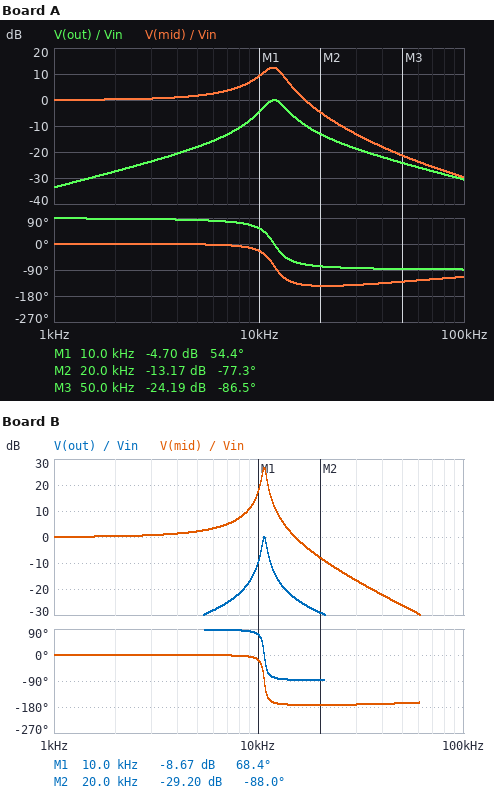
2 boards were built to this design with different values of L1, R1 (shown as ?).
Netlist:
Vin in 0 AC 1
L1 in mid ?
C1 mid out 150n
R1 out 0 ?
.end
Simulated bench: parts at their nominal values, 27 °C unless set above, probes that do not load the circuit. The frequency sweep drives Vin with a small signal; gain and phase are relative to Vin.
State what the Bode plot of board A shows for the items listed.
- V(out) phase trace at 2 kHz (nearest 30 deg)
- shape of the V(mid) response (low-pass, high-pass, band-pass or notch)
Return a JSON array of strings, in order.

["90 deg", "low-pass"]
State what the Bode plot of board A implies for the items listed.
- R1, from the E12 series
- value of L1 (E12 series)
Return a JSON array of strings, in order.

["22 Ω", "1.2 mH"]
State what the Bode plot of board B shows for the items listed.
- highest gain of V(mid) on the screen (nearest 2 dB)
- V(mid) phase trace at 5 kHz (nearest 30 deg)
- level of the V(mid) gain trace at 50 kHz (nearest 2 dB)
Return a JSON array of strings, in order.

["26 dB", "0 deg", "-26 dB"]
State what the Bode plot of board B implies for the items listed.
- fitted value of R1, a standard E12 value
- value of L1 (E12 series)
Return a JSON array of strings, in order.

["4.7 Ω", "1.5 mH"]
